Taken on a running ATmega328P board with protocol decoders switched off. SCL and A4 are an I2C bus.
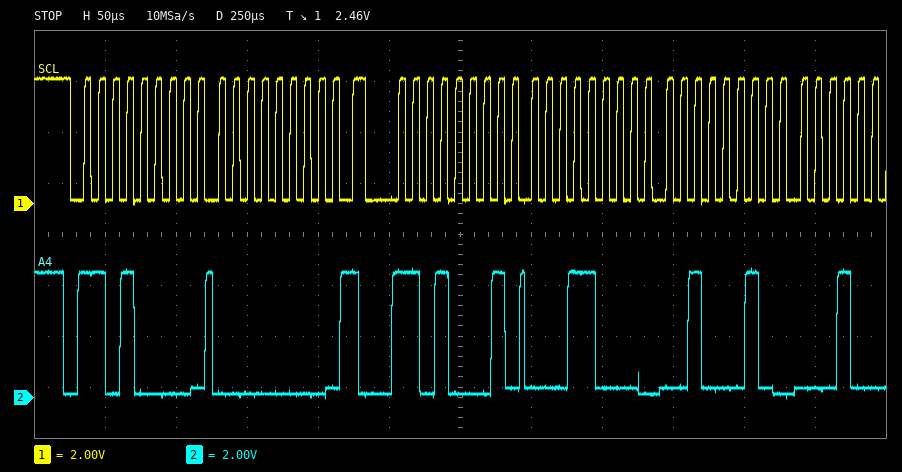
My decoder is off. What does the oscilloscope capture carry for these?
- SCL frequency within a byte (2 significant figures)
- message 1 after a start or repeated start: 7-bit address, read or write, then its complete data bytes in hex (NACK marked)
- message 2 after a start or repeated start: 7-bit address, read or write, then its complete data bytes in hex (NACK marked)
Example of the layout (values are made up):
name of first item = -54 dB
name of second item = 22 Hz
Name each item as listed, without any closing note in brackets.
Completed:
SCL frequency within a byte = 100 kHz
message 1 after a start or repeated start: 7-bit address, read or write, then its complete data bytes in hex = 0x68 write: 00
message 2 after a start or repeated start: 7-bit address, read or write, then its complete data bytes in hex = 0x68 read: 18 22
